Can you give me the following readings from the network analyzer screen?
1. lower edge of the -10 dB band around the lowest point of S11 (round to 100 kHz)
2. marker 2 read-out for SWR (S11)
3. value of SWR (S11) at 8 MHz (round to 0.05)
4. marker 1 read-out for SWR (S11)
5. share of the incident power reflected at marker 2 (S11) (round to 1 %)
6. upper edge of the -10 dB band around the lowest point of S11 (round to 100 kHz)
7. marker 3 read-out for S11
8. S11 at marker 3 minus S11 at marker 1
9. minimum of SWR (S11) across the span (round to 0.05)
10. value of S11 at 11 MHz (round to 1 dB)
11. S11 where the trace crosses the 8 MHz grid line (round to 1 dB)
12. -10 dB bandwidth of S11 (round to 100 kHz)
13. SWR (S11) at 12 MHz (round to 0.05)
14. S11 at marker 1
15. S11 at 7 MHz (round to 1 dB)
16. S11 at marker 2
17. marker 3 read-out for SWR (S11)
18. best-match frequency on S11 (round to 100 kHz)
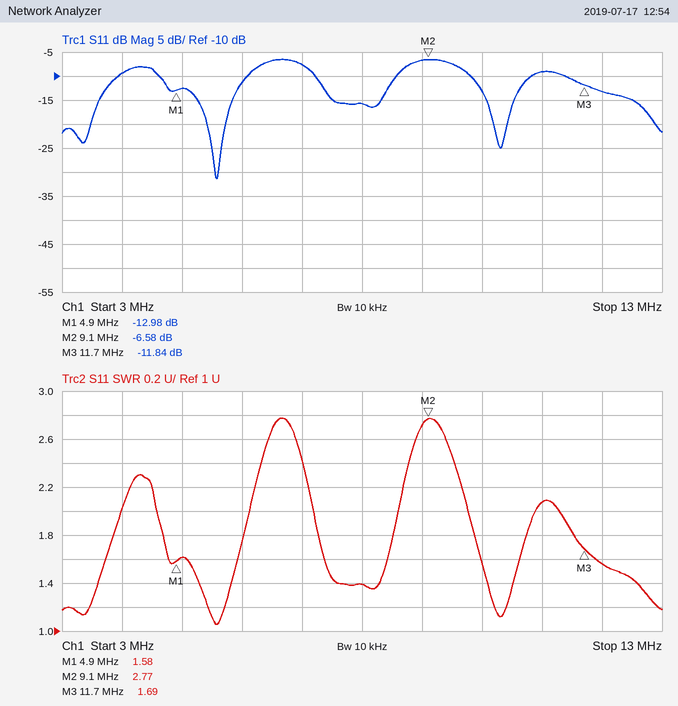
4.6 MHz
2.77
1.40
1.58
22 %
6.1 MHz
-11.84 dB
1.14 dB
1.05
-9 dB
-16 dB
1.5 MHz
1.55
-12.98 dB
-8 dB
-6.58 dB
1.69
5.6 MHz
